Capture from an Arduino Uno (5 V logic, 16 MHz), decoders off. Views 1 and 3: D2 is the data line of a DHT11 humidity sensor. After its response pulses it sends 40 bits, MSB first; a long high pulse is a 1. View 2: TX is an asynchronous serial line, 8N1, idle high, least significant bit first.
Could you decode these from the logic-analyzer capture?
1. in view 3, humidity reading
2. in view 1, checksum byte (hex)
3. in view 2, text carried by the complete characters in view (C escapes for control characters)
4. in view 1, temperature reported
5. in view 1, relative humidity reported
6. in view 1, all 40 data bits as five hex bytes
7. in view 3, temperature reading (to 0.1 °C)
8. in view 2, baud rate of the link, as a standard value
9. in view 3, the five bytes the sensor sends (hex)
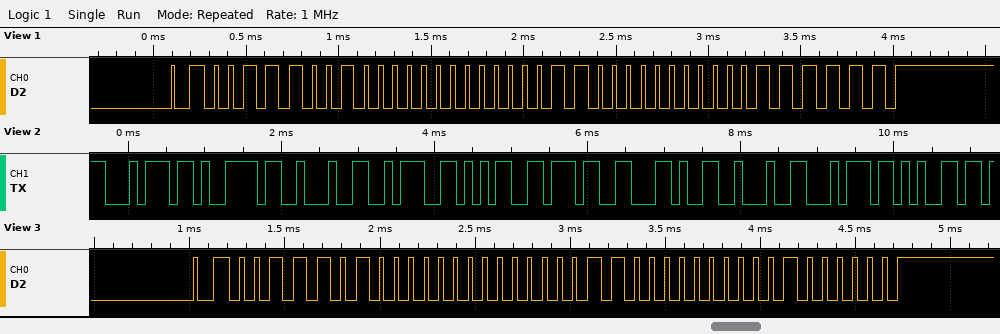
58 %
0x3F
"ty\":57,\"te"
6.0 °C
57 %
39 00 06 00 3F
6.0 °C
9600 baud
3A 00 06 00 40
